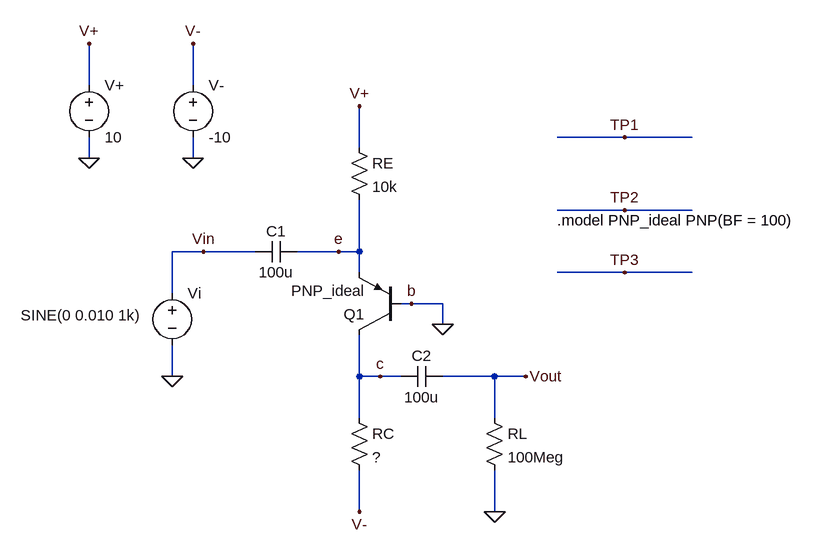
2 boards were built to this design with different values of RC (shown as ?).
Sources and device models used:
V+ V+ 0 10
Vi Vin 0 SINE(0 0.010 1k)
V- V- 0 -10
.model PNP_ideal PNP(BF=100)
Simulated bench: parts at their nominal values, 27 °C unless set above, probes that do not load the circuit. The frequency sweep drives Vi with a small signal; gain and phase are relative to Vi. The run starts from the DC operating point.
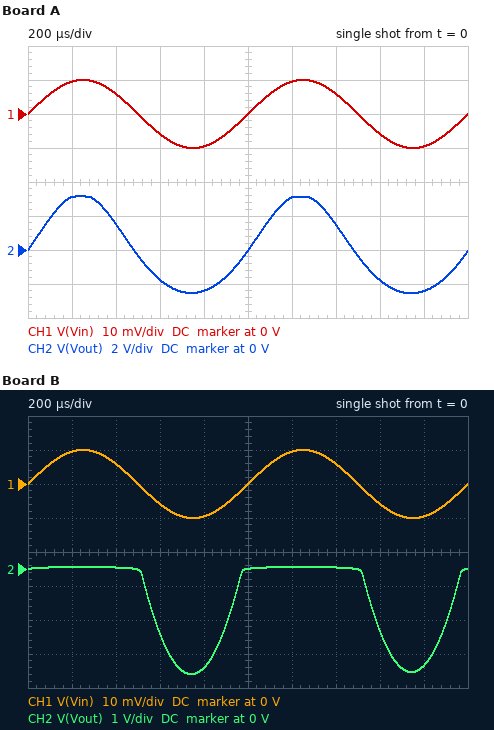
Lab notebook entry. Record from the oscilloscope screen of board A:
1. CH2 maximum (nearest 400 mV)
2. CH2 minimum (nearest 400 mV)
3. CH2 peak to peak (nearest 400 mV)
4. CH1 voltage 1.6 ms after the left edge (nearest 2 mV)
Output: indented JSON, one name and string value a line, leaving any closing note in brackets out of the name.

{
  "CH2 maximum": "3.2 V",
  "CH2 minimum": "-2.4 V",
  "CH2 peak to peak": "5.6 V",
  "CH1 voltage 1.6 ms after the left edge": "-6 mV"
}
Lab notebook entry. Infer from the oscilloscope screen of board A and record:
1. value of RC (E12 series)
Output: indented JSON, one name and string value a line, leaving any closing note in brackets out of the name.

{
  "value of RC": "8.2 kΩ"
}
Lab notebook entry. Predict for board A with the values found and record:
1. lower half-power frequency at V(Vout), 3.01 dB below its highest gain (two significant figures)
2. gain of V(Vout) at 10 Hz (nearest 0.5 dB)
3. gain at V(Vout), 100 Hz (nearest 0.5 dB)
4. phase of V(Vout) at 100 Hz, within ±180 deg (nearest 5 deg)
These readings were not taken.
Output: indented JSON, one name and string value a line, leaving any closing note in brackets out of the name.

{
  "lower half-power frequency at V(Vout), 3.01 dB below its highest gain": "57 Hz",
  "gain of V(Vout) at 10 Hz": "34.0 dB",
  "gain at V(Vout), 100 Hz": "48.0 dB",
  "phase of V(Vout) at 100 Hz, within ±180 deg": "30 deg"
}
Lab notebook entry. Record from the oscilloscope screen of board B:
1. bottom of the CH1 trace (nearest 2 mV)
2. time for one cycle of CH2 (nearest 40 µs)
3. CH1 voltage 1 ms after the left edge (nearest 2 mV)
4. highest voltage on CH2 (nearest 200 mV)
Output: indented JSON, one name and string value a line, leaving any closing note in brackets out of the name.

{
  "bottom of the CH1 trace": "-10 mV",
  "time for one cycle of CH2": "1.00 ms",
  "CH1 voltage 1 ms after the left edge": "0 V",
  "highest voltage on CH2": "0 V"
}
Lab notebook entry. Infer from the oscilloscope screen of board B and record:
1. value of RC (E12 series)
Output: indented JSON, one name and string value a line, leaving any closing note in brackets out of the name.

{
  "value of RC": "12 kΩ"
}
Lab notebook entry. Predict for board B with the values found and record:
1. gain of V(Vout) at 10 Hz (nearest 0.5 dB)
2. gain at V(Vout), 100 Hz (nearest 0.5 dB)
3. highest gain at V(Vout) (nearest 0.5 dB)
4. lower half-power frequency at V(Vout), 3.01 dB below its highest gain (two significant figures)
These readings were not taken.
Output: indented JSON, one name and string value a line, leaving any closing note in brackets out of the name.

{
  "gain of V(Vout) at 10 Hz": "15.5 dB",
  "gain at V(Vout), 100 Hz": "25.0 dB",
  "highest gain at V(Vout)": "25.5 dB",
  "lower half-power frequency at V(Vout), 3.01 dB below its highest gain": "31 Hz"
}
